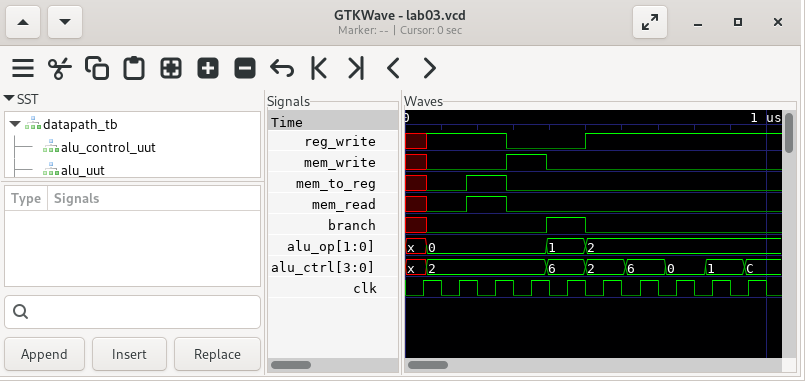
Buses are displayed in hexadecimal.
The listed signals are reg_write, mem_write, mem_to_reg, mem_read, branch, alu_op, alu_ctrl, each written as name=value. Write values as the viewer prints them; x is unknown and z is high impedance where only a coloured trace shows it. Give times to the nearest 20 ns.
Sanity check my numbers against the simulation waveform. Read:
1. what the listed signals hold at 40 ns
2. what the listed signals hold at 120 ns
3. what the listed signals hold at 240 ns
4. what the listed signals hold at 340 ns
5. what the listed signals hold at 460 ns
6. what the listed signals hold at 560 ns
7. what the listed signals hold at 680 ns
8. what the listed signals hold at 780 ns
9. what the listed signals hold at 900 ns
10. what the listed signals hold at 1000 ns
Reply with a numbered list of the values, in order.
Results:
1. reg_write=x, mem_write=x, mem_to_reg=x, mem_read=x, branch=x, alu_op=x, alu_ctrl=x
2. reg_write=1, mem_write=0, mem_to_reg=0, mem_read=0, branch=0, alu_op=0, alu_ctrl=2
3. reg_write=1, mem_write=0, mem_to_reg=1, mem_read=1, branch=0, alu_op=0, alu_ctrl=2
4. reg_write=0, mem_write=1, mem_to_reg=0, mem_read=0, branch=0, alu_op=0, alu_ctrl=2
5. reg_write=0, mem_write=0, mem_to_reg=0, mem_read=0, branch=1, alu_op=1, alu_ctrl=6
6. reg_write=1, mem_write=0, mem_to_reg=0, mem_read=0, branch=0, alu_op=2, alu_ctrl=2
7. reg_write=1, mem_write=0, mem_to_reg=0, mem_read=0, branch=0, alu_op=2, alu_ctrl=6
8. reg_write=1, mem_write=0, mem_to_reg=0, mem_read=0, branch=0, alu_op=2, alu_ctrl=0
9. reg_write=1, mem_write=0, mem_to_reg=0, mem_read=0, branch=0, alu_op=2, alu_ctrl=1
10. reg_write=1, mem_write=0, mem_to_reg=0, mem_read=0, branch=0, alu_op=2, alu_ctrl=C
